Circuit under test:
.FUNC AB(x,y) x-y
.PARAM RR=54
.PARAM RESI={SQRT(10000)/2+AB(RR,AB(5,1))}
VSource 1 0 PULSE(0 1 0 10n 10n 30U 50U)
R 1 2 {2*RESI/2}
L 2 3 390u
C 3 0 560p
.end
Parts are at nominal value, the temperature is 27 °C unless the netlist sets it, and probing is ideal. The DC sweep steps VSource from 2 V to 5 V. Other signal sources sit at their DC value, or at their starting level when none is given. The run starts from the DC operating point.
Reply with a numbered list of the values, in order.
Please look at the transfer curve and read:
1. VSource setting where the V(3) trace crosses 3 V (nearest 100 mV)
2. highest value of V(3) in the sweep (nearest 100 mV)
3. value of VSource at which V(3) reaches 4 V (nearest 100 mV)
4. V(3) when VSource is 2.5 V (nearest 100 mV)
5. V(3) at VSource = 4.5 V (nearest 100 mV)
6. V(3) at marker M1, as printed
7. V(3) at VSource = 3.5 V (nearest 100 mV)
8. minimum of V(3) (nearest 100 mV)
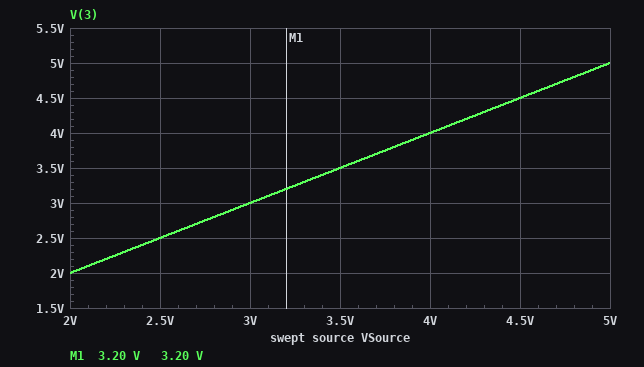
1. 3.0 V
2. 5.0 V
3. 4.0 V
4. 2.5 V
5. 4.5 V
6. 3.20 V
7. 3.5 V
8. 2.0 V
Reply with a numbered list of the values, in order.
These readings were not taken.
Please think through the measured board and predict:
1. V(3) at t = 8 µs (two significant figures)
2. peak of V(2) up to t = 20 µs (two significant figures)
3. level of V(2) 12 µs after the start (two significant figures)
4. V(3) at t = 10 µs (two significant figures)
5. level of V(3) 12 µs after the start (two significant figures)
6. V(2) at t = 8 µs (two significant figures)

1. 1.1 V
2. 1.1 V
3. 990 mV
4. 1.2 V
5. 800 mV
6. 1.0 V
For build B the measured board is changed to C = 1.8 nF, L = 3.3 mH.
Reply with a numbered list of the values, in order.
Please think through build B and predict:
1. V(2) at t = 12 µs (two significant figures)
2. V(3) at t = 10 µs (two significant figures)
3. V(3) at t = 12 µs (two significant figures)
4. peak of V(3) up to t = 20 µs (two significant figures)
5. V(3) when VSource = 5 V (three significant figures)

1. 1.1 V
2. 1.5 V
3. 860 mV
4. 1.9 V
5. 5.00 V
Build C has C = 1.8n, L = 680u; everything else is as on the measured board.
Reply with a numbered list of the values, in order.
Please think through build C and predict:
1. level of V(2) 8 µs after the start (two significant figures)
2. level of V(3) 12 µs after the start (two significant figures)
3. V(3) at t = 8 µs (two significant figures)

1. 930 mV
2. 1.1 V
3. 630 mV
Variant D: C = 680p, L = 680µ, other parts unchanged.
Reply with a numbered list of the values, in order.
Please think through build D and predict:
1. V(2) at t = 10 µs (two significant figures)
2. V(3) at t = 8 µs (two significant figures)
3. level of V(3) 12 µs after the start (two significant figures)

1. 960 mV
2. 640 mV
3. 880 mV
